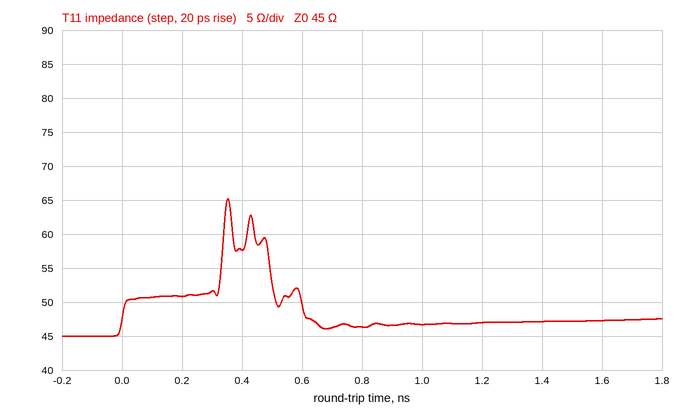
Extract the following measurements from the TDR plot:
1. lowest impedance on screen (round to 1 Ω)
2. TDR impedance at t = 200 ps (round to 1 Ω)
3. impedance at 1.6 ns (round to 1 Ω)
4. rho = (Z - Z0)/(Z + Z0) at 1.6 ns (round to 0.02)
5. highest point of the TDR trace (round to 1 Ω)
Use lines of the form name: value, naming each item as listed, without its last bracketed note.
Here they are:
lowest impedance on screen: 45 Ω
TDR impedance at t = 200 ps: 51 Ω
impedance at 1.6 ns: 47 Ω
rho = (Z - Z0)/(Z + Z0) at 1.6 ns: +0.02
highest point of the TDR trace: 65 Ω
